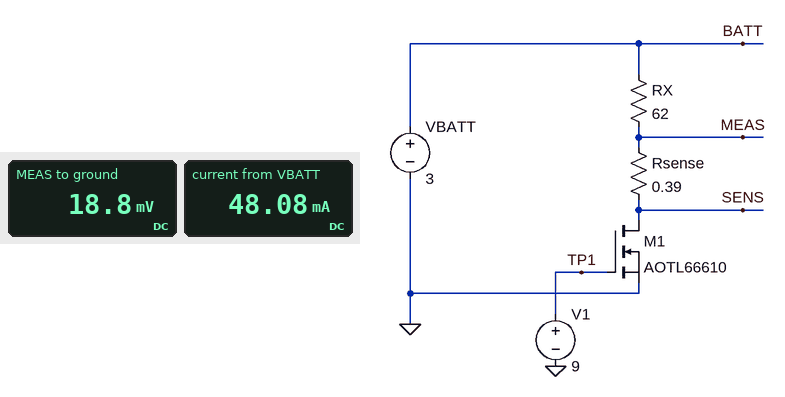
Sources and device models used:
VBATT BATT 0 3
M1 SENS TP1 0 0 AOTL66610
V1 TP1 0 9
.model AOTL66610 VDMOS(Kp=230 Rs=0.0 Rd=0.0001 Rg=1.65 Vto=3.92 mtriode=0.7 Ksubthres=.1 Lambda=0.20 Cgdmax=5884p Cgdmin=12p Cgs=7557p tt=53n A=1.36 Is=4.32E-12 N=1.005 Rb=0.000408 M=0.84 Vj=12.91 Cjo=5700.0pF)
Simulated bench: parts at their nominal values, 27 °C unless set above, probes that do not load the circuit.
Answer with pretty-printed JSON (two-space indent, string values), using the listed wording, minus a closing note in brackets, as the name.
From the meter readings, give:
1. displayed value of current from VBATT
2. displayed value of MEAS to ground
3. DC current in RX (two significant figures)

{
  "displayed value of current from VBATT": "48.08 mA",
  "displayed value of MEAS to ground": "18.8 mV",
  "DC current in RX": "48 mA"
}
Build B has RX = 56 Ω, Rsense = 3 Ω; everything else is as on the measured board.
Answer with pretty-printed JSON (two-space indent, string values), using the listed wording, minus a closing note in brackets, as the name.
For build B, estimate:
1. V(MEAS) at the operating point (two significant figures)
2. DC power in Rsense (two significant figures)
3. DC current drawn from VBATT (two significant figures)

{
  "V(MEAS) at the operating point": "150 mV",
  "DC power in Rsense": "7.8 mW",
  "DC current drawn from VBATT": "51 mA"
}
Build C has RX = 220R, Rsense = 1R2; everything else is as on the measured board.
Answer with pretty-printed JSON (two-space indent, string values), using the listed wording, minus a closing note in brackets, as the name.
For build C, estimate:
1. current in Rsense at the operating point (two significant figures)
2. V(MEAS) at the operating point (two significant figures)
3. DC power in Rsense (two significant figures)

{
  "current in Rsense at the operating point": "14 mA",
  "V(MEAS) at the operating point": "16 mV",
  "DC power in Rsense": "220 µW"
}
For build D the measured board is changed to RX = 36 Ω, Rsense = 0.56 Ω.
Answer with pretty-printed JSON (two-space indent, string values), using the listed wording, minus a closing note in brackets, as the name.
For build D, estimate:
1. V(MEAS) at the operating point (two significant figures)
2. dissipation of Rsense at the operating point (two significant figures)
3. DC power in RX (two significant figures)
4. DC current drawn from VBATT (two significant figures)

{
  "V(MEAS) at the operating point": "46 mV",
  "dissipation of Rsense at the operating point": "3.8 mW",
  "DC power in RX": "240 mW",
  "DC current drawn from VBATT": "82 mA"
}
